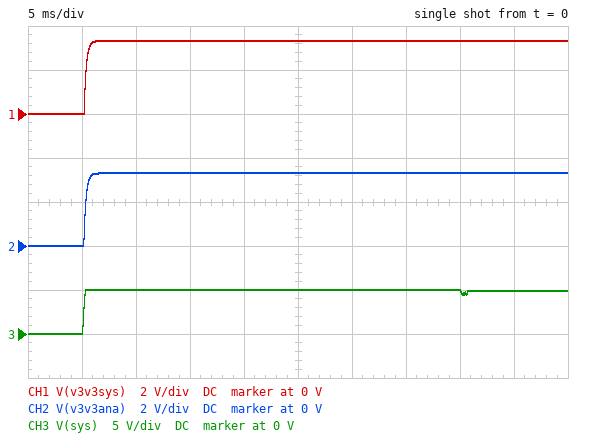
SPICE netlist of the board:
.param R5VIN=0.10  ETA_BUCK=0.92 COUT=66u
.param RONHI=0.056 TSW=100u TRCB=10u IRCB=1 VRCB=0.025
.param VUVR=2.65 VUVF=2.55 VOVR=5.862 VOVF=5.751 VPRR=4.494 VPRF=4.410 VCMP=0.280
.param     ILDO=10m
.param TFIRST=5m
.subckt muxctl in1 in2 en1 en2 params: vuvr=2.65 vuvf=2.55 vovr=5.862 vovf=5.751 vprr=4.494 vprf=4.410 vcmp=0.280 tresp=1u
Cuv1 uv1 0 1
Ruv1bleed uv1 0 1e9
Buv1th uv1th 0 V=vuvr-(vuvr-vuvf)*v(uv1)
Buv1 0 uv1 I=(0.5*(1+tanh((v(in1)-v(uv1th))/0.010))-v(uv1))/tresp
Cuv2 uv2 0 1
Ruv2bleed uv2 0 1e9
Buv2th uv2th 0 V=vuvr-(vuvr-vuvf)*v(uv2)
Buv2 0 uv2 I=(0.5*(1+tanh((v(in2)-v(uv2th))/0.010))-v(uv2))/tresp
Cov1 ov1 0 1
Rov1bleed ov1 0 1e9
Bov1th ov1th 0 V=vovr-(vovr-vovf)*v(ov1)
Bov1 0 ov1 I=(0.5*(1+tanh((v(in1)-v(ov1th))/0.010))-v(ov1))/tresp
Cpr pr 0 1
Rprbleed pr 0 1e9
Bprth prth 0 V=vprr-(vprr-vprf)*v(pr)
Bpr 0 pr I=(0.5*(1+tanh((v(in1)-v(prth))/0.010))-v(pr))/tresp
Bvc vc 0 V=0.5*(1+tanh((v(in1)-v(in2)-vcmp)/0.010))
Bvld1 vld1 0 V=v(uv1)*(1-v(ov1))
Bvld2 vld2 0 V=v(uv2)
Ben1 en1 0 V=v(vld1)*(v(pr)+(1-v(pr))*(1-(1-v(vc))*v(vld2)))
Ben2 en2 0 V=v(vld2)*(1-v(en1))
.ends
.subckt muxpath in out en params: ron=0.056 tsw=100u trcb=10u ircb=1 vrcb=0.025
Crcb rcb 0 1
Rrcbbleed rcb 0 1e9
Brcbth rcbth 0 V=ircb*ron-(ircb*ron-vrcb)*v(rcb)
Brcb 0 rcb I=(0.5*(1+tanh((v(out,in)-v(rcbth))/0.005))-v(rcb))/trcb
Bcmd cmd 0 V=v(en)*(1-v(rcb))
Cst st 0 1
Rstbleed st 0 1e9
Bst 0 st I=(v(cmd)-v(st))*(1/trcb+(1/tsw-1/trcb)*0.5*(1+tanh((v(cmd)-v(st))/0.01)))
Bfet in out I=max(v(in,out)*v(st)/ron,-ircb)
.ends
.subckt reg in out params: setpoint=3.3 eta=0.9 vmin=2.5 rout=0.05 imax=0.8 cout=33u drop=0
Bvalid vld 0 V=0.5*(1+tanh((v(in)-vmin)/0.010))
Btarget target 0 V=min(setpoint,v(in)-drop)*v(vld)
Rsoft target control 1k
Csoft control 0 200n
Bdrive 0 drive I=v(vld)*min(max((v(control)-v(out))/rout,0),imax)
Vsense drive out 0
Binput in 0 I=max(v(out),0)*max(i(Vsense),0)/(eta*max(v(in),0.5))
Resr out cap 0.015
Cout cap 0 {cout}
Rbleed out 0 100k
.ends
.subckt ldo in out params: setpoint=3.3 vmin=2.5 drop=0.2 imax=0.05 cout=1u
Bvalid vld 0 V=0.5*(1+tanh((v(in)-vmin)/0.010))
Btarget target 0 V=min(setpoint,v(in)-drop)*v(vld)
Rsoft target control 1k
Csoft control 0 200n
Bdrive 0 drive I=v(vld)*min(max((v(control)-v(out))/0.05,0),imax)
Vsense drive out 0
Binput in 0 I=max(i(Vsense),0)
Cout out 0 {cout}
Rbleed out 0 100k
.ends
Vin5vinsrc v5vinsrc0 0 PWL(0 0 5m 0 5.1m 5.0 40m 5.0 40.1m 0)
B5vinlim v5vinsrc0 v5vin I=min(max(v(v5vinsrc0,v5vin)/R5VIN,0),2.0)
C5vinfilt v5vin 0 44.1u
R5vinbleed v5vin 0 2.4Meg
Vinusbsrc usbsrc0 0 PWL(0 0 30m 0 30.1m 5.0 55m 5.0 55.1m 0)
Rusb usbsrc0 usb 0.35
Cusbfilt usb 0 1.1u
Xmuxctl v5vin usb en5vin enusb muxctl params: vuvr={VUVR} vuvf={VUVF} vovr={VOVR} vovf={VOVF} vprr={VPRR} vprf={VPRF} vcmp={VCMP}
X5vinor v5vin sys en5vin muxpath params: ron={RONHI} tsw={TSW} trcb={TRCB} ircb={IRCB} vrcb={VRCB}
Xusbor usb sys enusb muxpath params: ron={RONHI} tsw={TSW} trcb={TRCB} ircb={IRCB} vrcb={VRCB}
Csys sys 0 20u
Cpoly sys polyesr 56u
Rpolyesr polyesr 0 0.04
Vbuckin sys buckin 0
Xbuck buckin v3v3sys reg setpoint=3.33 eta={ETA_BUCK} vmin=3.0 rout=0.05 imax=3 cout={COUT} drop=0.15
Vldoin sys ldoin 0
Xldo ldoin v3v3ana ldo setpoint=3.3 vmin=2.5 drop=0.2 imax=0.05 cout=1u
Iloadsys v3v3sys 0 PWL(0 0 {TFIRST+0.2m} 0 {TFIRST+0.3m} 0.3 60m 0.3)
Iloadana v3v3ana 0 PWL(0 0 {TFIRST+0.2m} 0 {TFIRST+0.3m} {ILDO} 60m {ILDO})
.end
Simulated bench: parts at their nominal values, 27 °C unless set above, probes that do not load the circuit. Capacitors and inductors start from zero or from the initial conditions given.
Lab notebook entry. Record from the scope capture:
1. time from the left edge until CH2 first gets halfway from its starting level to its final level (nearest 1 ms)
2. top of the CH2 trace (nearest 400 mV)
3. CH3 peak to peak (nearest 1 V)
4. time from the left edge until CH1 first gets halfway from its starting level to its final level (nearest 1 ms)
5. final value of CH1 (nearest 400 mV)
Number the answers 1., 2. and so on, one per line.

1. 5 ms
2. 3.2 V
3. 5 V
4. 5 ms
5. 3.2 V
